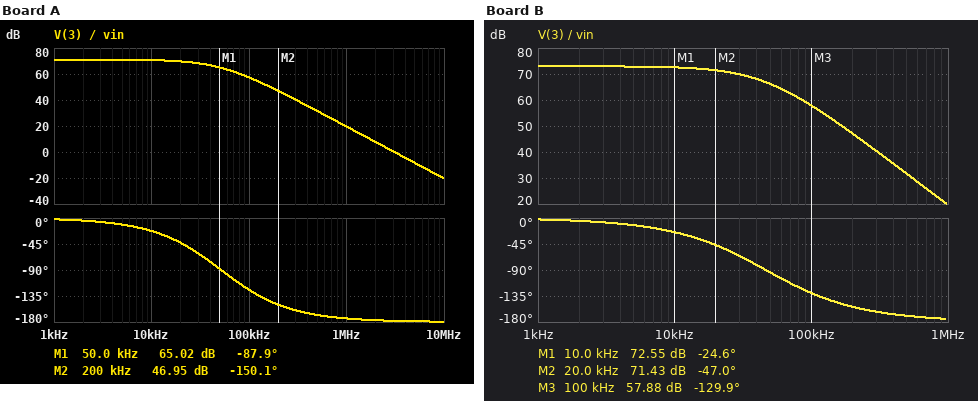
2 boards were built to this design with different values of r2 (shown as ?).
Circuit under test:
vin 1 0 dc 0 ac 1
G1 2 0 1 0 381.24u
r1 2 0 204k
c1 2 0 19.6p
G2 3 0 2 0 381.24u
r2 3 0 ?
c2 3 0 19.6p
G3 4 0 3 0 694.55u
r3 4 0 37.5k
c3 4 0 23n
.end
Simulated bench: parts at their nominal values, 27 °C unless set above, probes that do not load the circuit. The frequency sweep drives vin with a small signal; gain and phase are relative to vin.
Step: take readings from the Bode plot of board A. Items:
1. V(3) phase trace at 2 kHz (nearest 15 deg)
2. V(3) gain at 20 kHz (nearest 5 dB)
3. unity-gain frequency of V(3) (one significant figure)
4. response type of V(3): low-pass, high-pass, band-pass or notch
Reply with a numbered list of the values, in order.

1. 0 deg
2. 70 dB
3. 3 MHz
4. low-pass
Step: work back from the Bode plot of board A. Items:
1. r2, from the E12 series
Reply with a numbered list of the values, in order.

1. 120 kΩ
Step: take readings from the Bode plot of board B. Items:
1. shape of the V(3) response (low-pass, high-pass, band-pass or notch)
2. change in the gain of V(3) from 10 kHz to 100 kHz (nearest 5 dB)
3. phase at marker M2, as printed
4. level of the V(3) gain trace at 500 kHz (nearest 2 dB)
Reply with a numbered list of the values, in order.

1. low-pass
2. -15 dB
3. -47.0 deg
4. 32 dB
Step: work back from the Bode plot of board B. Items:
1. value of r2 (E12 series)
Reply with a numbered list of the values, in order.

1. 150 kΩ
